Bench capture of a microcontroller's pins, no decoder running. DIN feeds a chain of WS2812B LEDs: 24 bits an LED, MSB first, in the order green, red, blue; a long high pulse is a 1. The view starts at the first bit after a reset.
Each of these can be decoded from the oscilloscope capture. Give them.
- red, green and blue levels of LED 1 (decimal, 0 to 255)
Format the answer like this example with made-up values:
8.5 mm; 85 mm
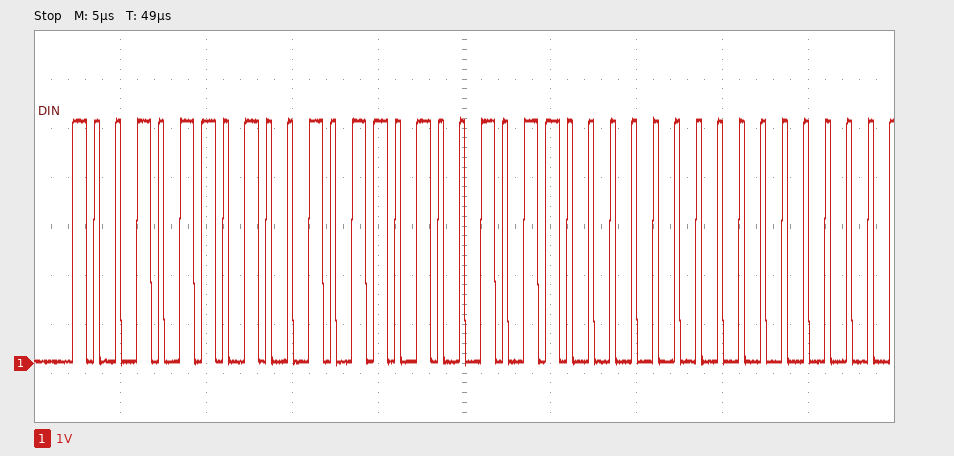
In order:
150, 150, 150
